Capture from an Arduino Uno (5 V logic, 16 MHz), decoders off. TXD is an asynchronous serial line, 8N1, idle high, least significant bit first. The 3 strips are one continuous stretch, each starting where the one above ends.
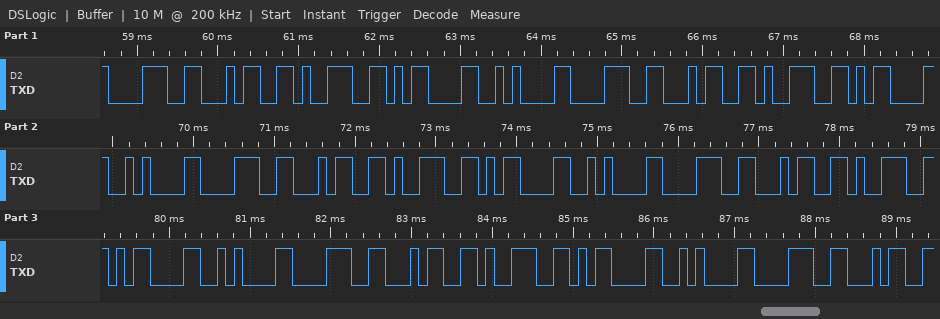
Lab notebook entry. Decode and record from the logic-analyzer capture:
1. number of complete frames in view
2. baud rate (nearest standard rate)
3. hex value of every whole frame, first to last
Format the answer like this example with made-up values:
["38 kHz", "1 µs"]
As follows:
["27", "9600 baud", "0x38 0x34 0x39 0x0D 0x0A 0x38 0x34 0x39 0x0D 0x0A 0x38 0x34 0x39 0x0D 0x0A 0x38 0x34 0x39 0x0D 0x0A 0x38 0x34 0x39 0x0D 0x0A 0x38 0x34"]
